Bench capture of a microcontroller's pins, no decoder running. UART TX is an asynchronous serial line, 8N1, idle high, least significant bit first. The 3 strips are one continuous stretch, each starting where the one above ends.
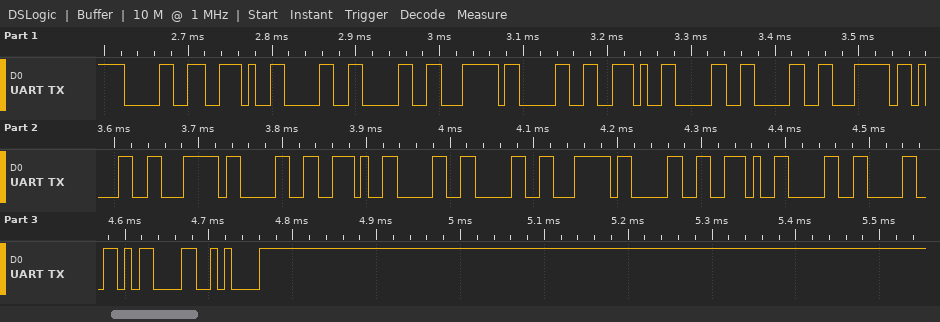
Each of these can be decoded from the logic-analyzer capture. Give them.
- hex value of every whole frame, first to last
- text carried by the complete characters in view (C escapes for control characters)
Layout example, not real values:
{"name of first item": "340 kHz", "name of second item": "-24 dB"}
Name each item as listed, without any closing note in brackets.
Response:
{"hex value of every whole frame, first to last": "0x30 0x2E 0x30 0x30 0x7C 0x30 0x2E 0x30 0x30 0x7C 0x31 0x7C 0x30 0x2E 0x30 0x30 0x7C 0x30 0x2E 0x30 0x30 0x0D 0x0A", "text carried by the complete characters in view": "\"0.00|0.00|1|0.00|0.00\\r\\n\""}
